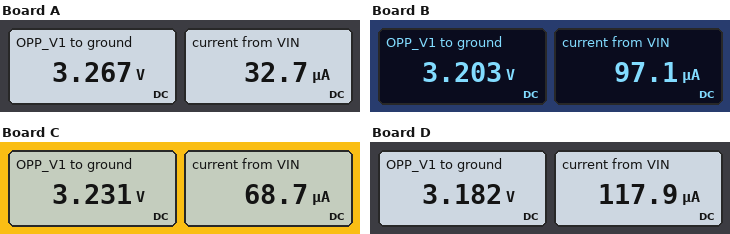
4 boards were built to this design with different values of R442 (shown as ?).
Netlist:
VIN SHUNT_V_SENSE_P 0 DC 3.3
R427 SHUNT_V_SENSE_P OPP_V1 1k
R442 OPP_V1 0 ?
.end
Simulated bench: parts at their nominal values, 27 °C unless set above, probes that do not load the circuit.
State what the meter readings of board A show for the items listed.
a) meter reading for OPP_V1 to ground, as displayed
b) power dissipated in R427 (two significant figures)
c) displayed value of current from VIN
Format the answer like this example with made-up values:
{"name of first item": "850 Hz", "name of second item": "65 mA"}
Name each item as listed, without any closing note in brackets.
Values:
{"meter reading for OPP_V1 to ground, as displayed": "3.267 V", "power dissipated in R427": "1.1 µW", "displayed value of current from VIN": "32.7 µA"}
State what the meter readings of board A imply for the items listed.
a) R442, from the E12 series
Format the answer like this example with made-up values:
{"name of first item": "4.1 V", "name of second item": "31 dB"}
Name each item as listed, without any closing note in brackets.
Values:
{"R442, from the E12 series": "100 kΩ"}
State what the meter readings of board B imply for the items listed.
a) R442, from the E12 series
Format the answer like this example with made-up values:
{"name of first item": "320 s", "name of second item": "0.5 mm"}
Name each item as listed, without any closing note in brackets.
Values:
{"R442, from the E12 series": "33 kΩ"}
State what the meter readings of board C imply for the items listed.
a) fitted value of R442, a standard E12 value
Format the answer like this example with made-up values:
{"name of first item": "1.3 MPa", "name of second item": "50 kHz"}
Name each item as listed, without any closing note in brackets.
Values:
{"fitted value of R442, a standard E12 value": "47 kΩ"}
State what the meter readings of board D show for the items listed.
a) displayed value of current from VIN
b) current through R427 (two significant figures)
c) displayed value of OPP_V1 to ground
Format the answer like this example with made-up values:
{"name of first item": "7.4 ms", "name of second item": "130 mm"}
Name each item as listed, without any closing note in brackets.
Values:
{"displayed value of current from VIN": "117.9 µA", "current through R427": "120 µA", "displayed value of OPP_V1 to ground": "3.182 V"}
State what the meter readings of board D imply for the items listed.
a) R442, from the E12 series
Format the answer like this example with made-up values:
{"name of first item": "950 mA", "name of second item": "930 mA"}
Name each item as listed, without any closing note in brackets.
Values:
{"R442, from the E12 series": "27 kΩ"}
